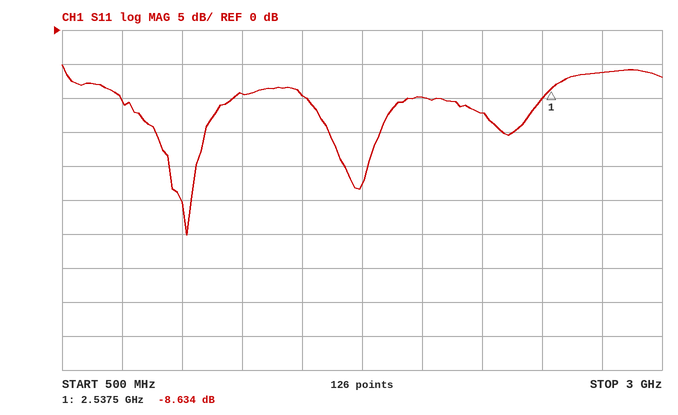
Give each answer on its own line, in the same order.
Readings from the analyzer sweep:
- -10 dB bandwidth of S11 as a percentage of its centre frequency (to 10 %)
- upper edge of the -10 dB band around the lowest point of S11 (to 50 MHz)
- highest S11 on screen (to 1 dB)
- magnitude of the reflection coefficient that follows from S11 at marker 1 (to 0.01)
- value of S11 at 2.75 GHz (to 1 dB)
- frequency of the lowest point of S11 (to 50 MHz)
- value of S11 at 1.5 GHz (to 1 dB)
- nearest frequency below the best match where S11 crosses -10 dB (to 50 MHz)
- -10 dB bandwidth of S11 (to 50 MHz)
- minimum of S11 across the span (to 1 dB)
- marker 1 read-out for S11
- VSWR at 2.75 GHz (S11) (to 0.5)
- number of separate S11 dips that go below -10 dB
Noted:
50 %
1.20 GHz
-5 dB
0.37
-6 dB
1.00 GHz
-10 dB
750 MHz
450 MHz
-30 dB
-8.634 dB
3.0
3
